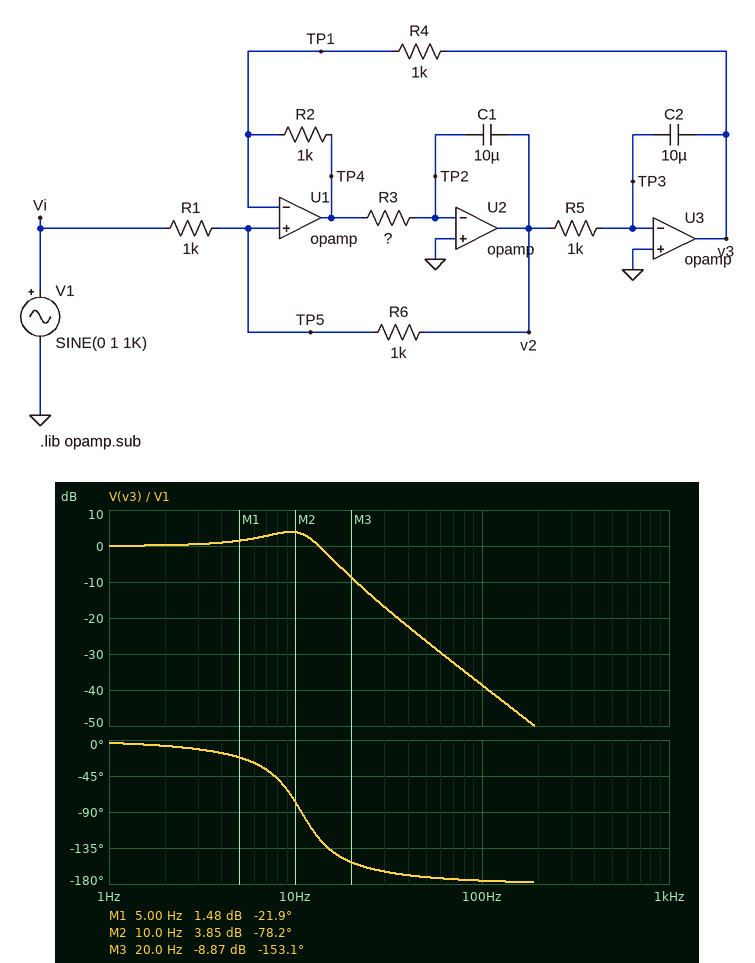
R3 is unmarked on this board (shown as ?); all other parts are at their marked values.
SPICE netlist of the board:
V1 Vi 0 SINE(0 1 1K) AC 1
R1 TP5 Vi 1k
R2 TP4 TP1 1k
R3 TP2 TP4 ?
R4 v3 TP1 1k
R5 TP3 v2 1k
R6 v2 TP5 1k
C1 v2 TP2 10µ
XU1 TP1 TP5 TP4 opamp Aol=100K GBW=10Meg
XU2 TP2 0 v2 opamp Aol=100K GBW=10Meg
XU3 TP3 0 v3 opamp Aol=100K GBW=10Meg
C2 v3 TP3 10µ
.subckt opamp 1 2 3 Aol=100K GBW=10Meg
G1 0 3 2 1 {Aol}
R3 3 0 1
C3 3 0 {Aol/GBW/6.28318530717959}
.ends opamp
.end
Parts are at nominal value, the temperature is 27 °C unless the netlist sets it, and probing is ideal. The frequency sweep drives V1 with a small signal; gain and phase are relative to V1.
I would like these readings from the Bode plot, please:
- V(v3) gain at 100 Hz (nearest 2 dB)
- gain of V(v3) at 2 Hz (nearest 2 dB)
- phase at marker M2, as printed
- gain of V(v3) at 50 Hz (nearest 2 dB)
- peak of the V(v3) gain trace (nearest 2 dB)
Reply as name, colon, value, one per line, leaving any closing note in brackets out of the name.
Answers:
V(v3) gain at 100 Hz: -38 dB
gain of V(v3) at 2 Hz: 0 dB
phase at marker M2, as printed: -78.2 deg
gain of V(v3) at 50 Hz: -26 dB
peak of the V(v3) gain trace: 4 dB
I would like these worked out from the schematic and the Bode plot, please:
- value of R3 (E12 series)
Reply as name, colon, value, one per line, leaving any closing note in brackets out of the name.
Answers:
value of R3: 2.2 kΩ
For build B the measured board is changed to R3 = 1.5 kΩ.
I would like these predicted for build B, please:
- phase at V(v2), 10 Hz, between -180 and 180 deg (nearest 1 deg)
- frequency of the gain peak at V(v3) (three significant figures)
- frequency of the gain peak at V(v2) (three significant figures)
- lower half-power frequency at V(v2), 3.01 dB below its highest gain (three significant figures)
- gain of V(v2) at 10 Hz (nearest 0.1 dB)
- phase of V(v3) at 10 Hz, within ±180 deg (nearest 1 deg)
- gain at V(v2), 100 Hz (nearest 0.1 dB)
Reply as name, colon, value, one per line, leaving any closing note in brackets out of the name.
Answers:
phase at V(v2), 10 Hz, between -180 and 180 deg: -147 deg
frequency of the gain peak at V(v3): 10.6 Hz
frequency of the gain peak at V(v2): 13.0 Hz
lower half-power frequency at V(v2), 3.01 dB below its highest gain: 8.73 Hz
gain of V(v2) at 10 Hz: -1.5 dB
phase of V(v3) at 10 Hz, within ±180 deg: -57 deg
gain at V(v2), 100 Hz: -19.4 dB
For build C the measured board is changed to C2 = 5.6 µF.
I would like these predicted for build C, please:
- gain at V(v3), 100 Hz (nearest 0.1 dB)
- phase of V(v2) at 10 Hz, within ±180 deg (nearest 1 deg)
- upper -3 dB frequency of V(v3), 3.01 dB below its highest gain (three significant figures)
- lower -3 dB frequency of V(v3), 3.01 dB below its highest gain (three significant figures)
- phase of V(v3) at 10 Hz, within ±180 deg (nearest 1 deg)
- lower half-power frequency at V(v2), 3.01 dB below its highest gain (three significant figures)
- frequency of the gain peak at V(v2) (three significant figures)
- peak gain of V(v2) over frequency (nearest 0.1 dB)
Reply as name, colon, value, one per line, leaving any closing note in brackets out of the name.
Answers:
gain at V(v3), 100 Hz: -33.6 dB
phase of V(v2) at 10 Hz, within ±180 deg: -124 deg
upper -3 dB frequency of V(v3), 3.01 dB below its highest gain: 16.7 Hz
lower -3 dB frequency of V(v3), 3.01 dB below its highest gain: 8.89 Hz
phase of V(v3) at 10 Hz, within ±180 deg: -34 deg
lower half-power frequency at V(v2), 3.01 dB below its highest gain: 11.2 Hz
frequency of the gain peak at V(v2): 14.3 Hz
peak gain of V(v2) over frequency: 0 dB
